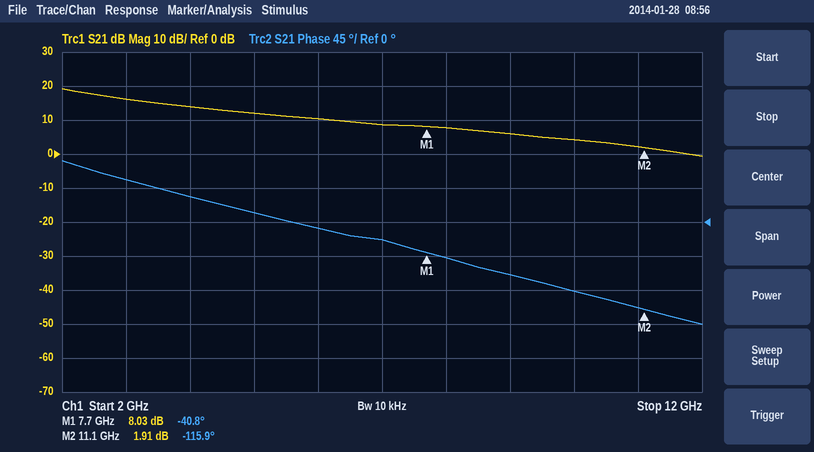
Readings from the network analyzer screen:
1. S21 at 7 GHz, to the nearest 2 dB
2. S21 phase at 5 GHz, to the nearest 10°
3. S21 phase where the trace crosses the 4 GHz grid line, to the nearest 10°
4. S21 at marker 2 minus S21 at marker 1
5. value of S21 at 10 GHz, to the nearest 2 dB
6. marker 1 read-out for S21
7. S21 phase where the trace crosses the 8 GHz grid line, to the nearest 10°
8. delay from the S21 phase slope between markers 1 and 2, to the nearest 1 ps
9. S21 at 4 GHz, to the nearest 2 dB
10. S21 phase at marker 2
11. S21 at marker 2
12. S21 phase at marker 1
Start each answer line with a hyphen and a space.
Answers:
- 8 dB
- 10°
- 30°
- -6.12 dB
- 4 dB
- 8.03 dB
- -50°
- 61 ps
- 14 dB
- -115.9°
- 1.91 dB
- -40.8°
